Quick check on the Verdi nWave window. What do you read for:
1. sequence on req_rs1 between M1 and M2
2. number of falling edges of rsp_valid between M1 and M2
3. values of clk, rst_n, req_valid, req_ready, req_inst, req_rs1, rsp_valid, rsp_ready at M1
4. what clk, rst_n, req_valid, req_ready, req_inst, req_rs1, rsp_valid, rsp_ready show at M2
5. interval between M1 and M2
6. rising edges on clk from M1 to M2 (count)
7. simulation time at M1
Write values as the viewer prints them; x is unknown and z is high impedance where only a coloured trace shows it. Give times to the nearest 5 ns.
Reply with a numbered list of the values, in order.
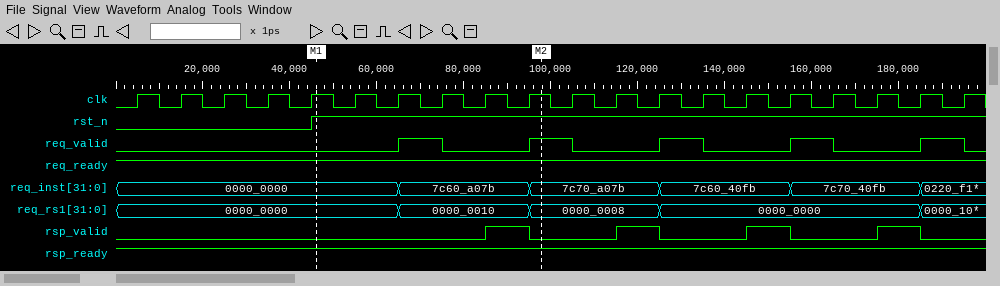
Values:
1. 0000_0000, 0000_0010, 0000_0008
2. 1
3. clk=1, rst_n=1, req_valid=0, req_ready=1, req_inst=0000_0000, req_rs1=0000_0000, rsp_valid=0, rsp_ready=1
4. clk=1, rst_n=1, req_valid=1, req_ready=1, req_inst=7c70_a07b, req_rs1=0000_0008, rsp_valid=0, rsp_ready=1
5. 50 ns
6. 5
7. 45 ns
